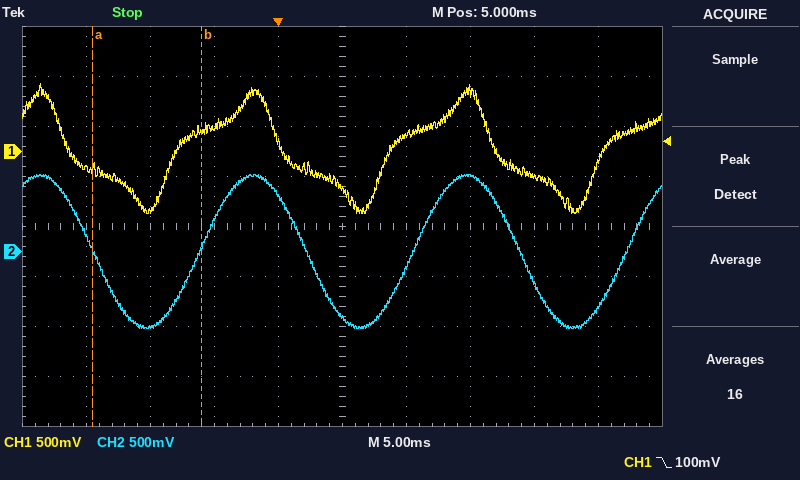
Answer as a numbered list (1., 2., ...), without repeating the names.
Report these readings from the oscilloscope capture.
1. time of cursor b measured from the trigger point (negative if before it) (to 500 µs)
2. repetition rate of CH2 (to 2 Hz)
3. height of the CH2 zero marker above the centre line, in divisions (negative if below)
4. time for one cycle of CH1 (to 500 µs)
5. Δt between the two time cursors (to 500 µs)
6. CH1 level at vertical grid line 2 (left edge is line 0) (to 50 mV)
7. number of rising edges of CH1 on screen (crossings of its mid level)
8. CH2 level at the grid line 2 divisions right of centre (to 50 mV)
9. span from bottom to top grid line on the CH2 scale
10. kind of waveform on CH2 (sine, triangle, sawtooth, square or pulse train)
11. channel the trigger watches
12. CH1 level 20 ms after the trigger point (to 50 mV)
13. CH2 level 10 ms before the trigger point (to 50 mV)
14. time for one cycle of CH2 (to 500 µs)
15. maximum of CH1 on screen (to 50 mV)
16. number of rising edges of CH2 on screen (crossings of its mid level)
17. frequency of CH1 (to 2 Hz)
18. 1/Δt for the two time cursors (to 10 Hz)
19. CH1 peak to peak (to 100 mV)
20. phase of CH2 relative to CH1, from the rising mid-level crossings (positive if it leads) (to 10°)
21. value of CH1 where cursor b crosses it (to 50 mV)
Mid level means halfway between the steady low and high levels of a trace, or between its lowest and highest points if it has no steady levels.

1. -6.0 ms
2. 60 Hz
3. -0.5 div
4. 16.5 ms
5. 8.5 ms
6. -600 mV
7. 3
8. 750 mV
9. 4 V
10. sine
11. CH1
12. -250 mV
13. -750 mV
14. 16.5 ms
15. 700 mV
16. 3
17. 60 Hz
18. 120 Hz
19. 1.30 V
20. -40°
21. 200 mV
